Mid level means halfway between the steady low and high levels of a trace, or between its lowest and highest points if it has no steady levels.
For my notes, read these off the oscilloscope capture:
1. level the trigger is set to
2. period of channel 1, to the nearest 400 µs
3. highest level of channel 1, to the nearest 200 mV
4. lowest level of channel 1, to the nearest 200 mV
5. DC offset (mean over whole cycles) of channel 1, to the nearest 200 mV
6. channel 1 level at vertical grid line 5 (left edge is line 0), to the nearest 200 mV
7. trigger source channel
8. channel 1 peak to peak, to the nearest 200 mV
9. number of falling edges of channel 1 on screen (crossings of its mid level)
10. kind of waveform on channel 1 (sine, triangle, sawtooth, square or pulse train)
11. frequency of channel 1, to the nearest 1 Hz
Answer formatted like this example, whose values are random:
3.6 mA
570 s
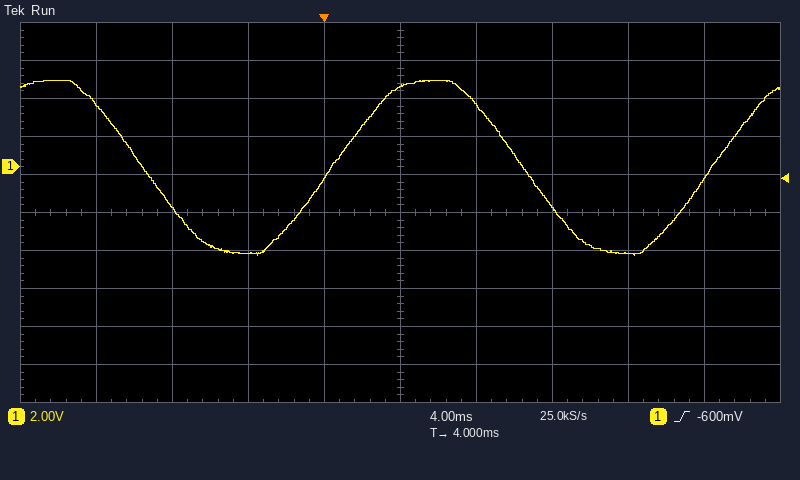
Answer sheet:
-600 mV
20.0 ms
4.6 V
-4.6 V
0.0 V
4.2 V
channel 1
9.2 V
2
sine
50 Hz
